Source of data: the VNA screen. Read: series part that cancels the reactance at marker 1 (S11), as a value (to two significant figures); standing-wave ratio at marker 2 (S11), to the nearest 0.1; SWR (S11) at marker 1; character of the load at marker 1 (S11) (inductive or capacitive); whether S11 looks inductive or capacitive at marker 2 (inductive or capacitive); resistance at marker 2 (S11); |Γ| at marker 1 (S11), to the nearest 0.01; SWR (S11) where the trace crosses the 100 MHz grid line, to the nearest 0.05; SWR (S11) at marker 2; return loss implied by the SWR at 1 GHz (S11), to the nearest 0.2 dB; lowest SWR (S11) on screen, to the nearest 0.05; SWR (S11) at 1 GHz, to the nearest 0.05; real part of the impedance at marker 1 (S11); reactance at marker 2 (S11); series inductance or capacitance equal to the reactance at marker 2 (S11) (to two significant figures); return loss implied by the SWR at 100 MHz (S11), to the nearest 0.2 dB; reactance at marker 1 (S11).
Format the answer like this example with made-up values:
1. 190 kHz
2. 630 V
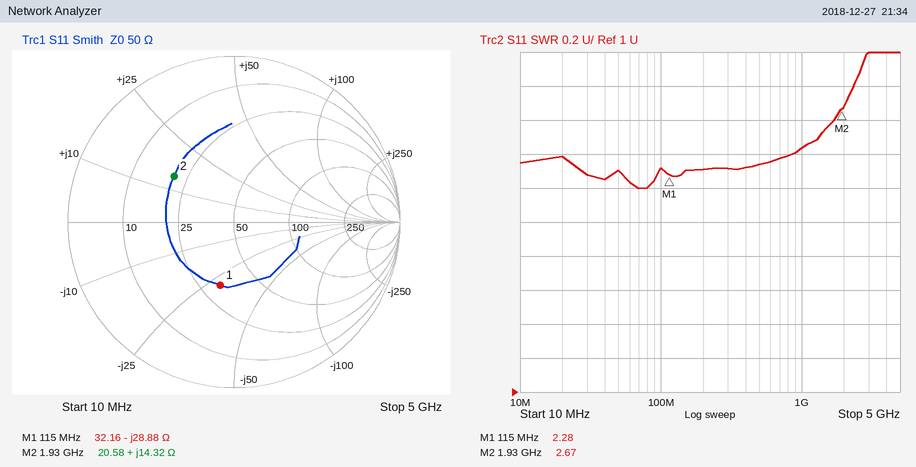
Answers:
1. 40 nH
2. 2.7
3. 2.28
4. capacitive
5. inductive
6. 20.58 Ω
7. 0.39
8. 2.30
9. 2.67
10. 7.6 dB
11. 2.20
12. 2.45
13. 32.16 Ω
14. +14.32 Ω
15. 1.2 nH
16. 8.0 dB
17. -28.88 Ω
